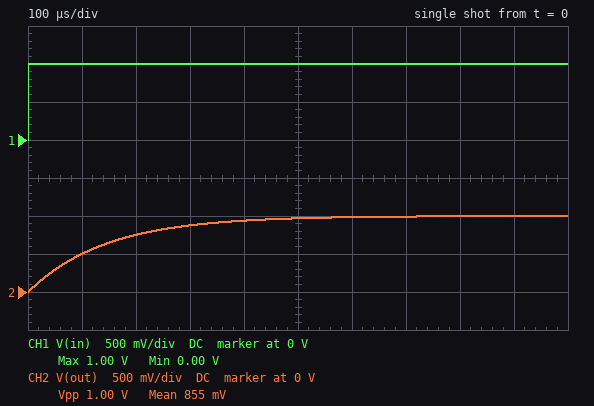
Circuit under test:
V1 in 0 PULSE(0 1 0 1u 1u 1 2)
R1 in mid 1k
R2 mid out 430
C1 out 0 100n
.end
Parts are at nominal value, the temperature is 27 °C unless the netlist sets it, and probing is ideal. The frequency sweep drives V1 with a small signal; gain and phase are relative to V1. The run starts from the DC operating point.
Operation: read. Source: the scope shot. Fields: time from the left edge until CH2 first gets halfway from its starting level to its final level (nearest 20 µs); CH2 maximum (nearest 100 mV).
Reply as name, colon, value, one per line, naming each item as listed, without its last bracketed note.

time from the left edge until CH2 first gets halfway from its starting level to its final level: 100 µs
CH2 maximum: 1.0 V
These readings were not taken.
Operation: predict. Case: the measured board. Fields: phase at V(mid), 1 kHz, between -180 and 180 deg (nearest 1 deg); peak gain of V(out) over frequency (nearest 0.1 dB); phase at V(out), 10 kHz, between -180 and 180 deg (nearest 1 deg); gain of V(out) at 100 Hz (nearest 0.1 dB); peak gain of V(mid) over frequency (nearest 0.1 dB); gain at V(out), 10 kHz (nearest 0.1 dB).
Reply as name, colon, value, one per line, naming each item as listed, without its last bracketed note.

phase at V(mid), 1 kHz, between -180 and 180 deg: -27 deg
peak gain of V(out) over frequency: 0 dB
phase at V(out), 10 kHz, between -180 and 180 deg: -84 deg
gain of V(out) at 100 Hz: 0 dB
peak gain of V(mid) over frequency: 0 dB
gain at V(out), 10 kHz: -19.1 dB
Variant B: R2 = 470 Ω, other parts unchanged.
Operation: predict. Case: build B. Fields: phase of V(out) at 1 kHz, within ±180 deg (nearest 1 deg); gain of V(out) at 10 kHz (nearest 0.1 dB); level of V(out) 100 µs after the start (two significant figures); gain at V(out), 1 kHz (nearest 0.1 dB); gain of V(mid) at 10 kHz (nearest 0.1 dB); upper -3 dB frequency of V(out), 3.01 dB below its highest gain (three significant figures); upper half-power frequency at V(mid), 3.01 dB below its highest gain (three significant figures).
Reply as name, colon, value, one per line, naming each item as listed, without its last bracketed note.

phase of V(out) at 1 kHz, within ±180 deg: -43 deg
gain of V(out) at 10 kHz: -19.4 dB
level of V(out) 100 µs after the start: 490 mV
gain at V(out), 1 kHz: -2.7 dB
gain of V(mid) at 10 kHz: -9.5 dB
upper -3 dB frequency of V(out), 3.01 dB below its highest gain: 1.08 kHz
upper half-power frequency at V(mid), 3.01 dB below its highest gain: 1.21 kHz
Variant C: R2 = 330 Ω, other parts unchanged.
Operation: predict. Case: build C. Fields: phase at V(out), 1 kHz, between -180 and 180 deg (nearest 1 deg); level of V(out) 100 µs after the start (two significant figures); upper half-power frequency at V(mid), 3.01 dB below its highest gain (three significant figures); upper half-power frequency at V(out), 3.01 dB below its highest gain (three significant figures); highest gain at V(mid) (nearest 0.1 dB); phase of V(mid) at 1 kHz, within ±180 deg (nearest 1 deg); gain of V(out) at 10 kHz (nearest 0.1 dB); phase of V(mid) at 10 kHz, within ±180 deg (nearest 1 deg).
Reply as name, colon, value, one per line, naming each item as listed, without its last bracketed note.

phase at V(out), 1 kHz, between -180 and 180 deg: -40 deg
level of V(out) 100 µs after the start: 530 mV
upper half-power frequency at V(mid), 3.01 dB below its highest gain: 1.28 kHz
upper half-power frequency at V(out), 3.01 dB below its highest gain: 1.20 kHz
highest gain at V(mid): 0 dB
phase of V(mid) at 1 kHz, within ±180 deg: -28 deg
gain of V(out) at 10 kHz: -18.5 dB
phase of V(mid) at 10 kHz, within ±180 deg: -19 deg
